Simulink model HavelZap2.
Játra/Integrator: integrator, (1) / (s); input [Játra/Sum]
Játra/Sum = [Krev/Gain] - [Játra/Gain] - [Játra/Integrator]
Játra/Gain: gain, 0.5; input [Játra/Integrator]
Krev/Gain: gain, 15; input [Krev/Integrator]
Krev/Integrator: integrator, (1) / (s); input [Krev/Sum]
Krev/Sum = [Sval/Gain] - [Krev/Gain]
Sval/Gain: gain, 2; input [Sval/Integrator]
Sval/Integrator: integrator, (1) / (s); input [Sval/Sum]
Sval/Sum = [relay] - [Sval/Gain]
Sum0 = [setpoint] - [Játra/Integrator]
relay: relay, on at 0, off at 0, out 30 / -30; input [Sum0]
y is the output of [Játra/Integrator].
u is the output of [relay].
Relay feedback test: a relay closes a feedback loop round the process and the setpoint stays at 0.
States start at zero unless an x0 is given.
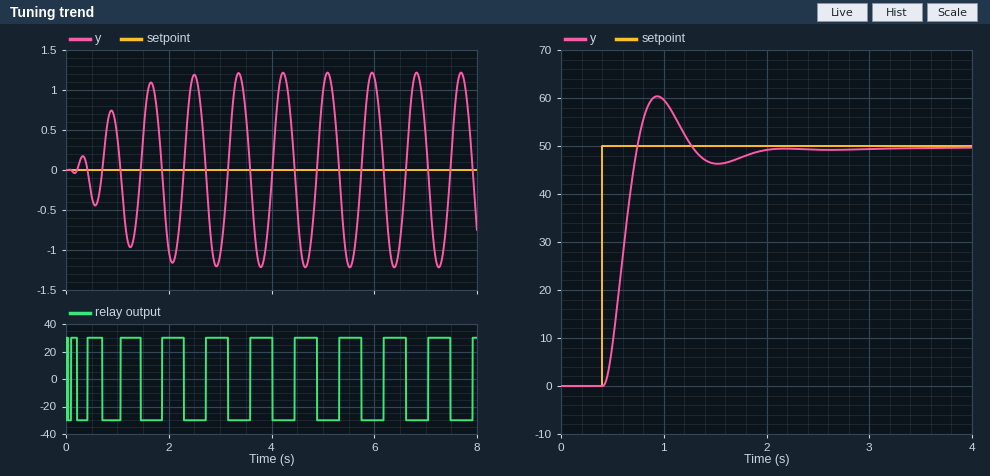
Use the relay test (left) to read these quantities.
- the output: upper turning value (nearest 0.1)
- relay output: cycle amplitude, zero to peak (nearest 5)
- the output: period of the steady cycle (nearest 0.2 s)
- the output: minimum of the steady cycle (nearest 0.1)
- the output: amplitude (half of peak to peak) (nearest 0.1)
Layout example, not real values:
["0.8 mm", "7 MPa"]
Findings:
["1.2", "30", "0.8 s", "-1.2", "1.2"]
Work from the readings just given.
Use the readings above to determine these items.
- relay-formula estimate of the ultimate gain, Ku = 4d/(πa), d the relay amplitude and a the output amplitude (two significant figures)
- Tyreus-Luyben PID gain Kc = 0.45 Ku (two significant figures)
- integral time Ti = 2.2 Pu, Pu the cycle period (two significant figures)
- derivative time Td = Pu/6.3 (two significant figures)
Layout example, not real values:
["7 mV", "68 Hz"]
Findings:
["32", "14", "1.8 s", "0.13 s"]
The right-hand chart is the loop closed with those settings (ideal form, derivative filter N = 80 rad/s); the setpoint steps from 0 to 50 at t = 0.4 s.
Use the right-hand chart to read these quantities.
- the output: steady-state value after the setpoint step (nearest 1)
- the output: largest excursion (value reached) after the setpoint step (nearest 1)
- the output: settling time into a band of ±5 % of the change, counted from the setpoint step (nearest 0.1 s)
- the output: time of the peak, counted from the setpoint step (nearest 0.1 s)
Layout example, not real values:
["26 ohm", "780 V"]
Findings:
["50", "60", "1.3 s", "0.5 s"]
